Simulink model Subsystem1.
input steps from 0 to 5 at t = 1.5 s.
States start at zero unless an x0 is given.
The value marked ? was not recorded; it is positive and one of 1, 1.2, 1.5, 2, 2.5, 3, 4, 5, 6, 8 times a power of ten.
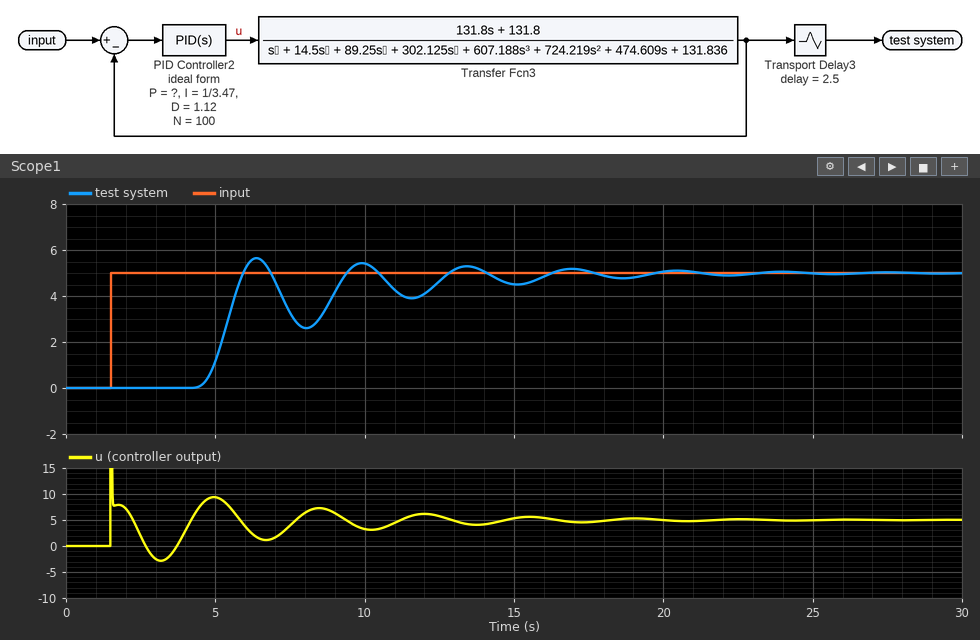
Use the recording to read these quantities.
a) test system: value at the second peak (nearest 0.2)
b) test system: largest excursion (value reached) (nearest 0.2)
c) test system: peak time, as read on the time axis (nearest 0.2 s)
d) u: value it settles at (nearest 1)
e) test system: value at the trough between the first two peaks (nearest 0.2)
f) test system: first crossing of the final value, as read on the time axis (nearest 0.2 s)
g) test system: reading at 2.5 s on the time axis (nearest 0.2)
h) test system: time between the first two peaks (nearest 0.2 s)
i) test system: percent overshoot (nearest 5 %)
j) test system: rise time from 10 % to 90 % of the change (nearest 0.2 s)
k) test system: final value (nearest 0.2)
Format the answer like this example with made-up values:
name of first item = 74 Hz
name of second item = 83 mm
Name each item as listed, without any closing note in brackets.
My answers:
test system: value at the second peak = 5.4
test system: largest excursion (value reached) = 5.6
test system: peak time, as read on the time axis = 6.4 s
u: value it settles at = 5
test system: value at the trough between the first two peaks = 2.6
test system: first crossing of the final value, as read on the time axis = 6.0 s
test system: reading at 2.5 s on the time axis = 0.0
test system: time between the first two peaks = 3.6 s
test system: percent overshoot = 15 %
test system: rise time from 10 % to 90 % of the change = 1.0 s
test system: final value = 5.0
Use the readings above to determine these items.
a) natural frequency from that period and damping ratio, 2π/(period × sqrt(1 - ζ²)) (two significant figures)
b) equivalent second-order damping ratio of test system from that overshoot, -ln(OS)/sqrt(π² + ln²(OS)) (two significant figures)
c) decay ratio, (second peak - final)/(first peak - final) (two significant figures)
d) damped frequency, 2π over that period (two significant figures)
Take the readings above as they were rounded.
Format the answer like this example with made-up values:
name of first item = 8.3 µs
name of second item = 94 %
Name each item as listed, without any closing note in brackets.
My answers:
natural frequency from that period and damping ratio, 2π/(period × sqrt(1 - ζ²)) = 2.0 rad/s
equivalent second-order damping ratio of test system from that overshoot, -ln(OS)/sqrt(π² + ln²(OS)) = 0.52
decay ratio, (second peak - final)/(first peak - final) = 0.67
damped frequency, 2π over that period = 1.7 rad/s
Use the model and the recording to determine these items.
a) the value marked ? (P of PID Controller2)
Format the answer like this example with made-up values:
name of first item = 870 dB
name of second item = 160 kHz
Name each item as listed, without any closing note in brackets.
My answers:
the value marked ? = 1.5
